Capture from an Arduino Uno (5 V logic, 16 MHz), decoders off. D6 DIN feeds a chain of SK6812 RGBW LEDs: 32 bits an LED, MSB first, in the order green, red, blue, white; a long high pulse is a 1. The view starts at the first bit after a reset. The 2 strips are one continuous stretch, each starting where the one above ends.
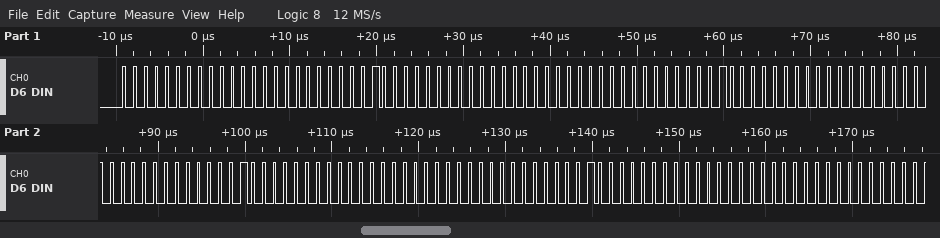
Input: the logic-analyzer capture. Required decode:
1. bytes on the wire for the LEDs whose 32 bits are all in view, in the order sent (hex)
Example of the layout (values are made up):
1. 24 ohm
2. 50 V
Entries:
1. 00 00 01 00 00 00 01 00 00 00 01 00 00 00 01 00
